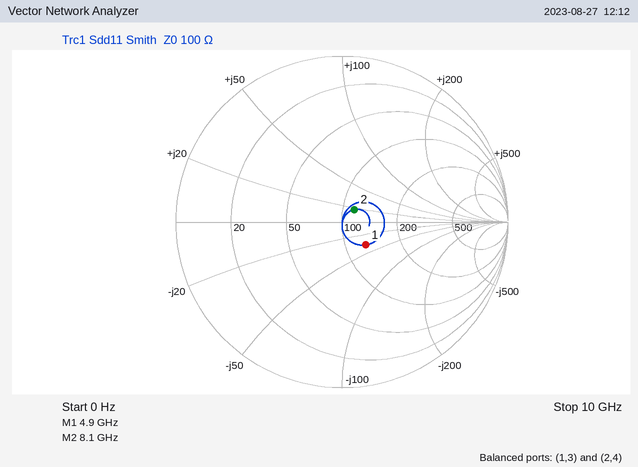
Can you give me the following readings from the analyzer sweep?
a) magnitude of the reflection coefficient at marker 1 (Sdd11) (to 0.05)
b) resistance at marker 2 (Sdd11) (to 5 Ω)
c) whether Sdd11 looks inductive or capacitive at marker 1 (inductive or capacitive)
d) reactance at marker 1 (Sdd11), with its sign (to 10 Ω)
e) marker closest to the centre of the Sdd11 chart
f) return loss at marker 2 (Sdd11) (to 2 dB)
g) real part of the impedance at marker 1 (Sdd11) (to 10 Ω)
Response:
0.20
115 Ω
capacitive
-40 Ω
marker 2
20 dB
130 Ω
